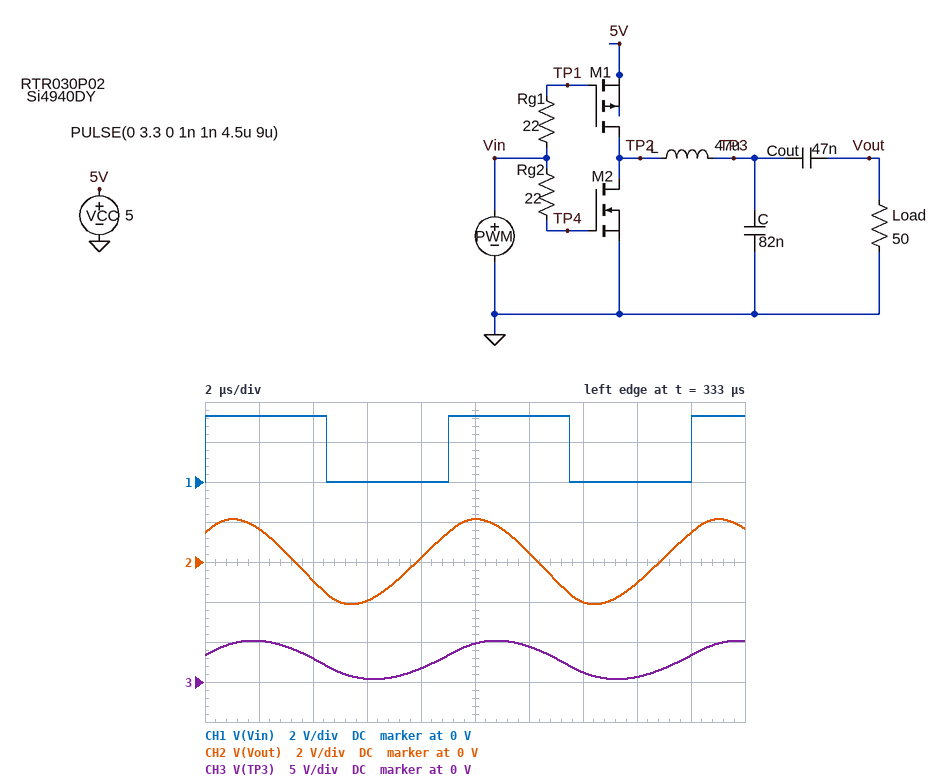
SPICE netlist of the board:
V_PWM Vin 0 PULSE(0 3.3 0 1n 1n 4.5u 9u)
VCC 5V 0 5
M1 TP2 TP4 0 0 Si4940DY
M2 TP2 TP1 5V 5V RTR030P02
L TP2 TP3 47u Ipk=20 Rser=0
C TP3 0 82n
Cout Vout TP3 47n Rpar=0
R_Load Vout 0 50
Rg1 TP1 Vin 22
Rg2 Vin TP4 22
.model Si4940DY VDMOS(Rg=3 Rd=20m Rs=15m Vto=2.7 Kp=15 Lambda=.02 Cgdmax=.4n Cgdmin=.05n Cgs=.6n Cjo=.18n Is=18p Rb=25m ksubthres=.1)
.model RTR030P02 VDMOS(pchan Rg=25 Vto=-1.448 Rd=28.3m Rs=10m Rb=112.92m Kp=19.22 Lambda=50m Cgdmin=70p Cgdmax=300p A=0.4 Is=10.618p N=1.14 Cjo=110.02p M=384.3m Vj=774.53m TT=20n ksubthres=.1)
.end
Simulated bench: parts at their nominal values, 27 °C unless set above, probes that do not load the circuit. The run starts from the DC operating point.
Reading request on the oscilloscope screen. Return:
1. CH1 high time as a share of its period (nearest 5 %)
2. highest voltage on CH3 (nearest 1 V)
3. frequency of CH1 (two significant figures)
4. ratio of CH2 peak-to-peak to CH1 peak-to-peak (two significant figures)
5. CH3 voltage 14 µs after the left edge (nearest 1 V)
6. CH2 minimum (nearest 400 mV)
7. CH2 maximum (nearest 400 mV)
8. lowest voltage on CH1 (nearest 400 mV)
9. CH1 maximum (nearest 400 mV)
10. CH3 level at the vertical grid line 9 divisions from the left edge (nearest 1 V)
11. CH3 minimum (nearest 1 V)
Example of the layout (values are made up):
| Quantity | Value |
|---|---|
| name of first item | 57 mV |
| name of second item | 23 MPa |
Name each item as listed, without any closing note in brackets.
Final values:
| Quantity | Value |
|---|---|
| CH1 high time as a share of its period | 50 % |
| highest voltage on CH3 | 5 V |
| frequency of CH1 | 110 kHz |
| ratio of CH2 peak-to-peak to CH1 peak-to-peak | 1.3 |
| CH3 voltage 14 µs after the left edge | 1 V |
| CH2 minimum | -2.0 V |
| CH2 maximum | 2.0 V |
| lowest voltage on CH1 | 0 V |
| CH1 maximum | 3.2 V |
| CH3 level at the vertical grid line 9 divisions from the left edge | 3 V |
| CH3 minimum | 0 V |
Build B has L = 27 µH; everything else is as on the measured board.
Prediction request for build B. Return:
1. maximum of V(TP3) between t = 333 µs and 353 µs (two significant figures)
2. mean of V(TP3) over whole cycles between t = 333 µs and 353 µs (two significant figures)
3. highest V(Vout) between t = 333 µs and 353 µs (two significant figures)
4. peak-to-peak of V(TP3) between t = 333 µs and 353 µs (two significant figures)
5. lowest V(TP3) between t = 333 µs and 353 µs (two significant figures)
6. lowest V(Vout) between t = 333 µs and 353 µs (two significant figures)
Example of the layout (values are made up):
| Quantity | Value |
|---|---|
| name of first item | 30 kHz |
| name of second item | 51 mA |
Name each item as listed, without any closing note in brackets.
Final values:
| Quantity | Value |
|---|---|
| maximum of V(TP3) between t = 333 µs and 353 µs | 11 V |
| mean of V(TP3) over whole cycles between t = 333 µs and 353 µs | 2.7 V |
| highest V(Vout) between t = 333 µs and 353 µs | 7.1 V |
| peak-to-peak of V(TP3) between t = 333 µs and 353 µs | 17 V |
| lowest V(TP3) between t = 333 µs and 353 µs | -5.6 V |
| lowest V(Vout) between t = 333 µs and 353 µs | -7.2 V |
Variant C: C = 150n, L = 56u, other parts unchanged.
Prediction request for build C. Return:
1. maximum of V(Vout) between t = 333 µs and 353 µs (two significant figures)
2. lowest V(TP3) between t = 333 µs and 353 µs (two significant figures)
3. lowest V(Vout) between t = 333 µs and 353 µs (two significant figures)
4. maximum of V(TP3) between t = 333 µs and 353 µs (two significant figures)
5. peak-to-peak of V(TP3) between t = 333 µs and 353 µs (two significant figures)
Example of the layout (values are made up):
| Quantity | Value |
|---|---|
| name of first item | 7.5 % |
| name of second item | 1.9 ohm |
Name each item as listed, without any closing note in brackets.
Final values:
| Quantity | Value |
|---|---|
| maximum of V(Vout) between t = 333 µs and 353 µs | 770 mV |
| lowest V(TP3) between t = 333 µs and 353 µs | 1.9 V |
| lowest V(Vout) between t = 333 µs and 353 µs | -750 mV |
| maximum of V(TP3) between t = 333 µs and 353 µs | 3.6 V |
| peak-to-peak of V(TP3) between t = 333 µs and 353 µs | 1.7 V |
